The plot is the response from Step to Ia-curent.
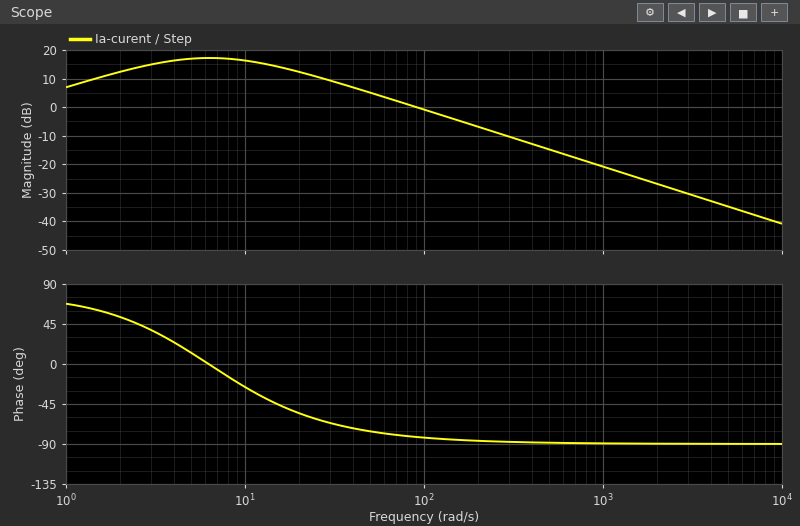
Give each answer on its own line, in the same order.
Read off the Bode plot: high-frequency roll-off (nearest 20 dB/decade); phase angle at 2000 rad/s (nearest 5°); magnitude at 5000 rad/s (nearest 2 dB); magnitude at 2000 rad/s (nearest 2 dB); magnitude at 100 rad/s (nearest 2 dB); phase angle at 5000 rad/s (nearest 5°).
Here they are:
-20 dB/decade
-90°
-34 dB
-26 dB
0 dB
-90°
